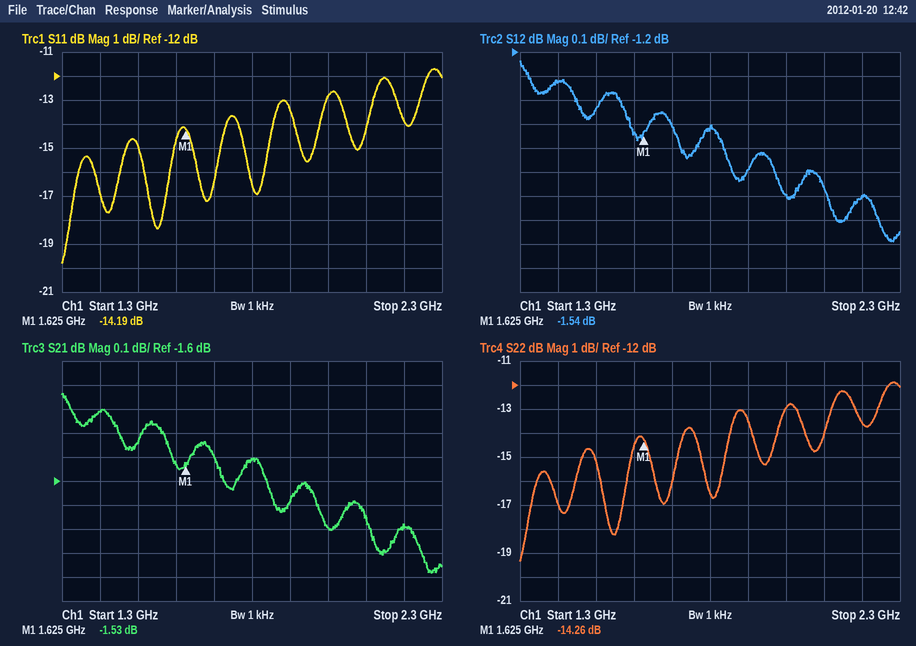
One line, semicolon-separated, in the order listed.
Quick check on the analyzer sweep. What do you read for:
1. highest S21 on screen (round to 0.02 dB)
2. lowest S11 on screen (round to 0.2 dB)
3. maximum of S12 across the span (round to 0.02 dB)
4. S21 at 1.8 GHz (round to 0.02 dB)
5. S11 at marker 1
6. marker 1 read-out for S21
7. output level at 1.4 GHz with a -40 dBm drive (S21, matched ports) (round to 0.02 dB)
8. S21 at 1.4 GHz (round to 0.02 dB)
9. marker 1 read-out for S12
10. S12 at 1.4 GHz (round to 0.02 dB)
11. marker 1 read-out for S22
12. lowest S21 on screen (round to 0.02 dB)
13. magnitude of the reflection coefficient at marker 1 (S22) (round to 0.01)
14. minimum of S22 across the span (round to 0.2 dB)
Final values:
-1.24 dB; -19.8 dB; -1.24 dB; -1.50 dB; -14.19 dB; -1.53 dB; -41.32 dBm; -1.32 dB; -1.54 dB; -1.32 dB; -14.26 dB; -1.98 dB; 0.19; -19.4 dB
